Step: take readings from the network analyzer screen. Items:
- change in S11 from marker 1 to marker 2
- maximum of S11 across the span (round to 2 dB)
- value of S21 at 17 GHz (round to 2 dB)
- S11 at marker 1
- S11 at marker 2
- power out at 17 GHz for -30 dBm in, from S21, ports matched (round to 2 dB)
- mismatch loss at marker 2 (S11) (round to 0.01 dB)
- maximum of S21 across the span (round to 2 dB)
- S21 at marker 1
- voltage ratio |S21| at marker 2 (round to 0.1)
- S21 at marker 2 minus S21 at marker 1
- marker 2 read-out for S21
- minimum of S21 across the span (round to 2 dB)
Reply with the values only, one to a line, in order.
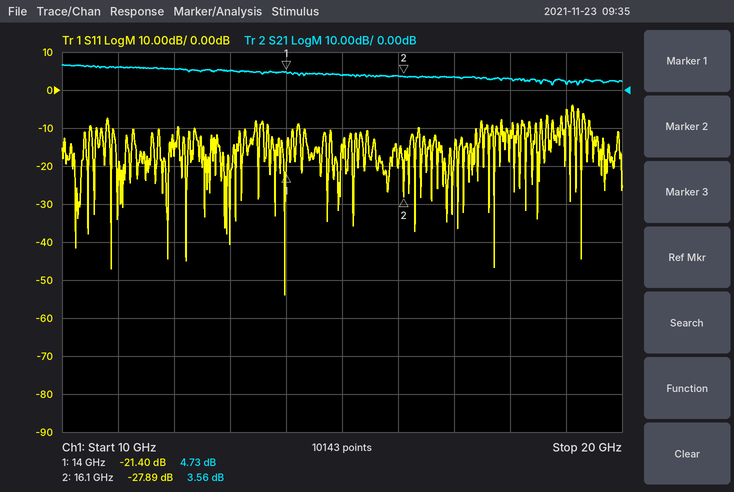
-6.49 dB
-4 dB
4 dB
-21.40 dB
-27.89 dB
-26 dBm
0.01 dB
6 dB
4.73 dB
1.5
-1.17 dB
3.56 dB
2 dB
